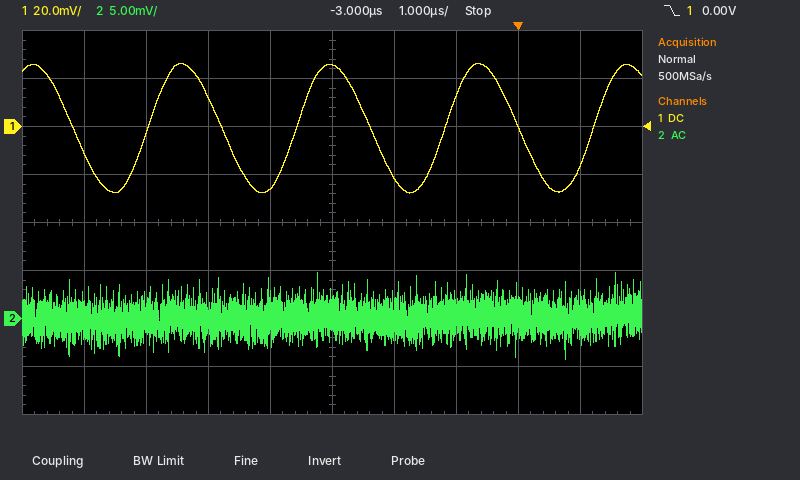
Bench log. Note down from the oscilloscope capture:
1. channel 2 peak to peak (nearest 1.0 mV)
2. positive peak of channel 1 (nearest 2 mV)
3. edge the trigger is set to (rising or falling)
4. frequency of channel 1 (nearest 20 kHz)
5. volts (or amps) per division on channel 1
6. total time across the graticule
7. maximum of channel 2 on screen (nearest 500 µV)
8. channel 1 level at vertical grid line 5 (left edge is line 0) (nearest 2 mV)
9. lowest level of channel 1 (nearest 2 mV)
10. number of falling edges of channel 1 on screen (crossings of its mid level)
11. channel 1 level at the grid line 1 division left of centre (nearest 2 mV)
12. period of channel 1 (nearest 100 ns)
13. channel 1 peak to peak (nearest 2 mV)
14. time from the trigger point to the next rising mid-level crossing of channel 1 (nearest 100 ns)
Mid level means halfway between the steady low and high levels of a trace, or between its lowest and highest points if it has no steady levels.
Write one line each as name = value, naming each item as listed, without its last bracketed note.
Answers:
channel 2 peak to peak = 9.0 mV
positive peak of channel 1 = 26 mV
edge the trigger is set to = falling
frequency of channel 1 = 420 kHz
volts (or amps) per division on channel 1 = 20 mV
total time across the graticule = 10 µs
maximum of channel 2 on screen = 5.0 mV
channel 1 level at vertical grid line 5 (left edge is line 0) = 26 mV
lowest level of channel 1 = -28 mV
number of falling edges of channel 1 on screen = 4
channel 1 level at the grid line 1 division left of centre = -26 mV
period of channel 1 = 2.4 µs
channel 1 peak to peak = 54 mV
time from the trigger point to the next rising mid-level crossing of channel 1 = 1.2 µs
